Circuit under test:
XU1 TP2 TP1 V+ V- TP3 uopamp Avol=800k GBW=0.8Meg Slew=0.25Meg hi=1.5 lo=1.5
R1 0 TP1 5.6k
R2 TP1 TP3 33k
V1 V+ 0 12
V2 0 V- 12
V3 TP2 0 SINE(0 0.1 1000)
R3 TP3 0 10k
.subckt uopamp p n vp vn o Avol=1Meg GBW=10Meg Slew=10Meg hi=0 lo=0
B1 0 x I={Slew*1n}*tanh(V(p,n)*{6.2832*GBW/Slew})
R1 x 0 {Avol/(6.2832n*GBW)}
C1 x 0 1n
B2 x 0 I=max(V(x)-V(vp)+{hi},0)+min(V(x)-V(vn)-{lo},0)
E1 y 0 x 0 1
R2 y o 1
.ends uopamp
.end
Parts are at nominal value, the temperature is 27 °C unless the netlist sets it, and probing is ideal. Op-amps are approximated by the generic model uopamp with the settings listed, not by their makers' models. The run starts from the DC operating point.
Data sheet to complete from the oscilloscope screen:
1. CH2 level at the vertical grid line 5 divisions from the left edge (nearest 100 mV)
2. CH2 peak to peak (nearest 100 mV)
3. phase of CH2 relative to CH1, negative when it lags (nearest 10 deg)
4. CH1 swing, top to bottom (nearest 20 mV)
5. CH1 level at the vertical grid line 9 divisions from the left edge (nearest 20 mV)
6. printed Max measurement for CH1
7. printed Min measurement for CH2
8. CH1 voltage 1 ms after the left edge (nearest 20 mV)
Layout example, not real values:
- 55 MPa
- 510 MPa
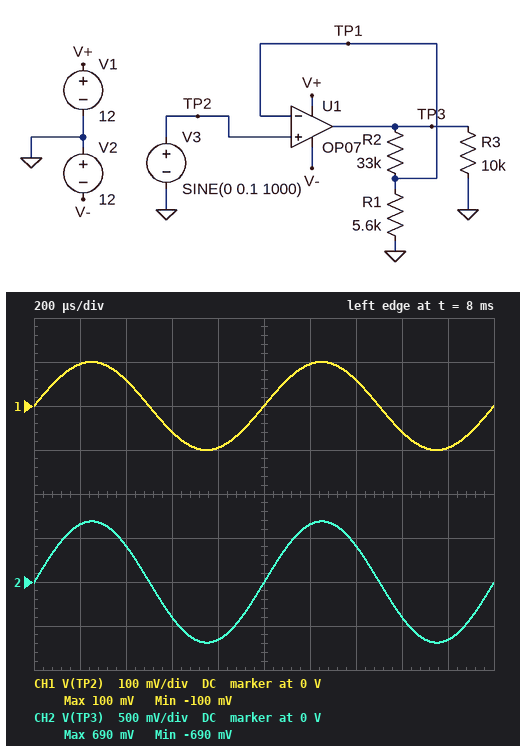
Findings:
- 0 V
- 1.4 V
- 0 deg
- 200 mV
- -100 mV
- 100 mV
- -690 mV
- 0 V
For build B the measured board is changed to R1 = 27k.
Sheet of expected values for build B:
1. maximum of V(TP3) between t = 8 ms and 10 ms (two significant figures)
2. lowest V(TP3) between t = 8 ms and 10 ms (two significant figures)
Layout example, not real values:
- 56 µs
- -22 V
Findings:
- 220 mV
- -220 mV
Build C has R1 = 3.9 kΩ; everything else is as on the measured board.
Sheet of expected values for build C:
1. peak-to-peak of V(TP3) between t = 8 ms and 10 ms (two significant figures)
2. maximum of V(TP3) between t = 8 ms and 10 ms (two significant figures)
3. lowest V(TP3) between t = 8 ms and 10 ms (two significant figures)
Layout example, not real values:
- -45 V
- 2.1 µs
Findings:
- 1.9 V
- 950 mV
- -950 mV
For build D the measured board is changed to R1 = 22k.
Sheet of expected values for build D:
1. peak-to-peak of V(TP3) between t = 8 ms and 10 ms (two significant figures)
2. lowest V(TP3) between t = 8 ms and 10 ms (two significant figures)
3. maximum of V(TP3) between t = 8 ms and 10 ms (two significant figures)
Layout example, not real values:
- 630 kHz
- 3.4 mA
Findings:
- 500 mV
- -250 mV
- 250 mV
